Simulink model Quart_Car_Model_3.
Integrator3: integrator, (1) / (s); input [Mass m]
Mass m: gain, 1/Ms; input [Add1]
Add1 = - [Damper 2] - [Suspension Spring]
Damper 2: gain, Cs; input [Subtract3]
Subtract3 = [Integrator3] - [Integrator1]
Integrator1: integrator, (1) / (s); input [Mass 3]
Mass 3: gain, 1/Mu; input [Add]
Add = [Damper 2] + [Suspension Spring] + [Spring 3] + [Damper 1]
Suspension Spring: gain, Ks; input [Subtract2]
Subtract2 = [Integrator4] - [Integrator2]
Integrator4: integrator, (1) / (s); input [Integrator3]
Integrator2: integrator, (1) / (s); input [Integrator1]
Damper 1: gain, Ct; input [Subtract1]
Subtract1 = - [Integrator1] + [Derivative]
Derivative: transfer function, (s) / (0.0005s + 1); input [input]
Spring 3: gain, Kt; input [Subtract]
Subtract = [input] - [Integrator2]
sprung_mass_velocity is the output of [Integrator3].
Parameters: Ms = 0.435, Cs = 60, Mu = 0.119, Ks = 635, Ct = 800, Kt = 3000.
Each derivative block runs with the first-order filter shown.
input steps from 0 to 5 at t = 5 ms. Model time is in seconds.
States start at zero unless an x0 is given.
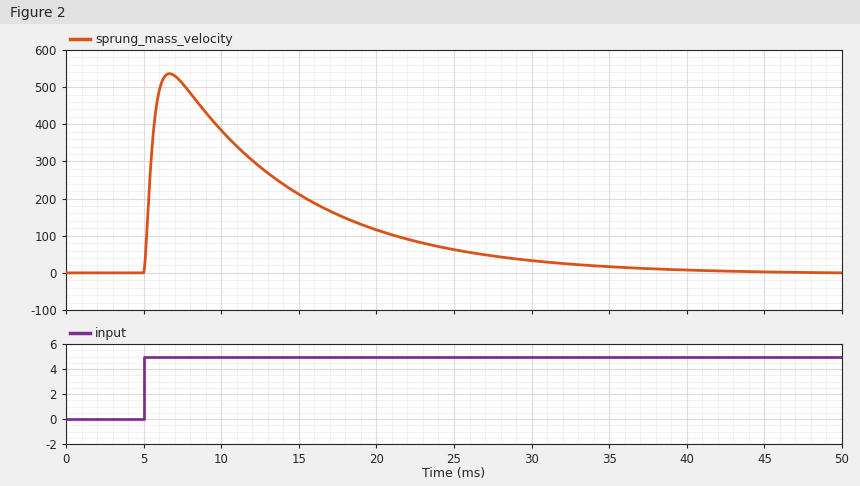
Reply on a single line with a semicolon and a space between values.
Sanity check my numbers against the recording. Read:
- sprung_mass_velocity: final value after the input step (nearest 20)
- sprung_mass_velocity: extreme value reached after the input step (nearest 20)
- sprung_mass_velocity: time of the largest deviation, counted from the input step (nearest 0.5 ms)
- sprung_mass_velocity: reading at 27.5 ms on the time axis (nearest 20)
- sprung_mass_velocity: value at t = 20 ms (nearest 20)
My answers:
0; 540; 1.5 ms; 40; 120
